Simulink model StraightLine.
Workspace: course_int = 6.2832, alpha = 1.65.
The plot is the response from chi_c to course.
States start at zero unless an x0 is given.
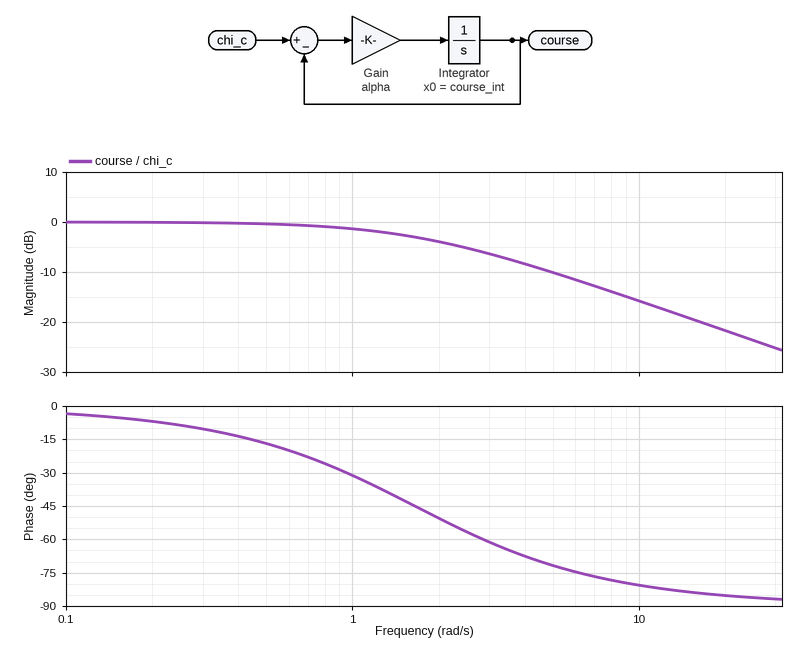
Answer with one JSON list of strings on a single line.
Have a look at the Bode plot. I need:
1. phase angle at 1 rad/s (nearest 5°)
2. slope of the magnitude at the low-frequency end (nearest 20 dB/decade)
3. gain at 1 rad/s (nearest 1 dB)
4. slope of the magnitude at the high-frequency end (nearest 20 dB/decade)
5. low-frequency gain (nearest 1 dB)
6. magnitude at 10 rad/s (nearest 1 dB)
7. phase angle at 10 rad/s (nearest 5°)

["-30°", "0 dB/decade", "-1 dB", "-20 dB/decade", "0 dB", "-16 dB", "-80°"]
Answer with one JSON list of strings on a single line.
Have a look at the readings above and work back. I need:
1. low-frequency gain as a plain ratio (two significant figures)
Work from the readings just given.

["1.0"]
